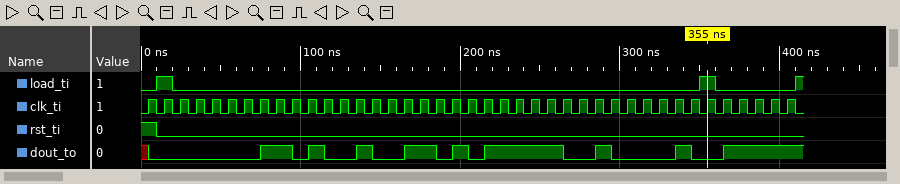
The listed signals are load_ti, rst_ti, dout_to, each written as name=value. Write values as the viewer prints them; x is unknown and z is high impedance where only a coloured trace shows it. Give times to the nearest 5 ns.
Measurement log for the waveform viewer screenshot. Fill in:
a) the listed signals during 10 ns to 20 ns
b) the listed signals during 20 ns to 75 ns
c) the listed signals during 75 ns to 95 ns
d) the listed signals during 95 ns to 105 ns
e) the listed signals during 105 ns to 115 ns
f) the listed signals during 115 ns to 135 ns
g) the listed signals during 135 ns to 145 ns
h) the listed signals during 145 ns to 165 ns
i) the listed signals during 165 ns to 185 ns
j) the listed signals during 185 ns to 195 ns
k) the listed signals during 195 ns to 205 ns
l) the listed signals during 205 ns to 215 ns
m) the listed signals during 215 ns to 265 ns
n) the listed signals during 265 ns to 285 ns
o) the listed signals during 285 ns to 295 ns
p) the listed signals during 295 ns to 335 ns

load_ti=1, rst_ti=0, dout_to=0
load_ti=0, rst_ti=0, dout_to=0
load_ti=0, rst_ti=0, dout_to=1
load_ti=0, rst_ti=0, dout_to=0
load_ti=0, rst_ti=0, dout_to=1
load_ti=0, rst_ti=0, dout_to=0
load_ti=0, rst_ti=0, dout_to=1
load_ti=0, rst_ti=0, dout_to=0
load_ti=0, rst_ti=0, dout_to=1
load_ti=0, rst_ti=0, dout_to=0
load_ti=0, rst_ti=0, dout_to=1
load_ti=0, rst_ti=0, dout_to=0
load_ti=0, rst_ti=0, dout_to=1
load_ti=0, rst_ti=0, dout_to=0
load_ti=0, rst_ti=0, dout_to=1
load_ti=0, rst_ti=0, dout_to=0
